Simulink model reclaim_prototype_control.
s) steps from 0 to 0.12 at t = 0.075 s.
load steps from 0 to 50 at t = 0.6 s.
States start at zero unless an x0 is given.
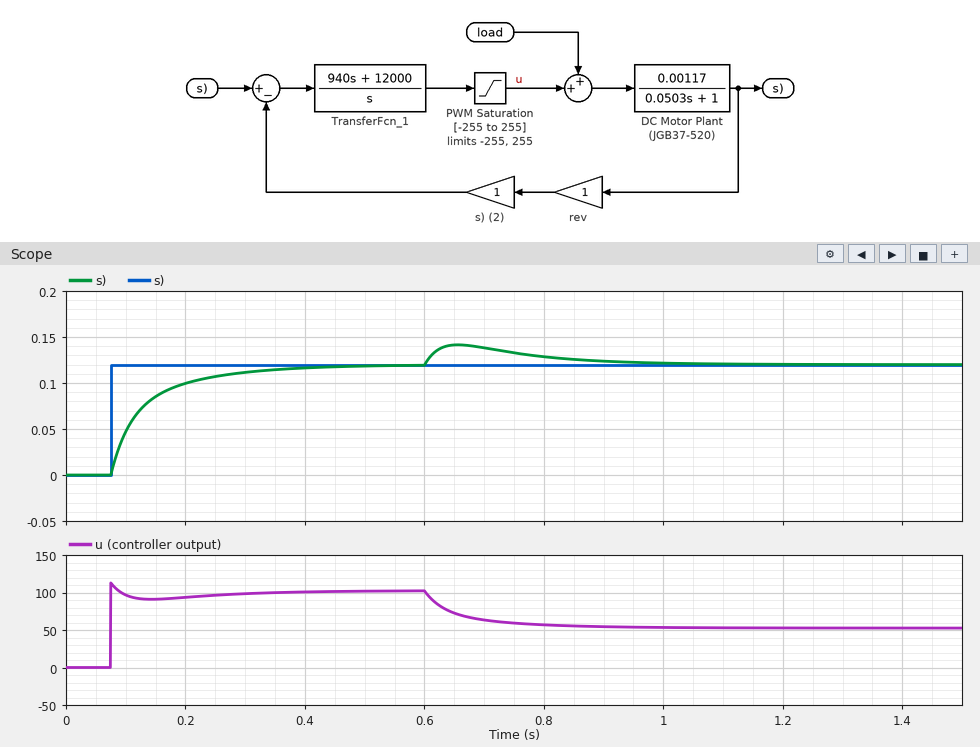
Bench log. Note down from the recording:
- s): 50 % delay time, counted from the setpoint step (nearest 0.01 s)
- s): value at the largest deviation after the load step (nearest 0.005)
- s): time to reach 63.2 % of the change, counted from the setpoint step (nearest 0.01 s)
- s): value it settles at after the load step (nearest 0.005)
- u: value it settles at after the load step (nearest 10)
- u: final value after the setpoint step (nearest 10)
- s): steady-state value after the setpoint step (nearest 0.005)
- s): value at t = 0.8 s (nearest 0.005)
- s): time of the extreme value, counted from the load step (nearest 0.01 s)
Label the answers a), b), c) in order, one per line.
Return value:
a) 0.04 s
b) 0.140
c) 0.06 s
d) 0.120
e) 50
f) 100
g) 0.120
h) 0.130
i) 0.06 s
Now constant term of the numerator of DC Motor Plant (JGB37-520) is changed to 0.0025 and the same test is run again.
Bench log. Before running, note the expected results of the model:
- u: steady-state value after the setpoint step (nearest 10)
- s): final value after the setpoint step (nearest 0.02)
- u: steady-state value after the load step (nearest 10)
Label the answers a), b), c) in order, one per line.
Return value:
a) 50
b) 0.12
c) 0
